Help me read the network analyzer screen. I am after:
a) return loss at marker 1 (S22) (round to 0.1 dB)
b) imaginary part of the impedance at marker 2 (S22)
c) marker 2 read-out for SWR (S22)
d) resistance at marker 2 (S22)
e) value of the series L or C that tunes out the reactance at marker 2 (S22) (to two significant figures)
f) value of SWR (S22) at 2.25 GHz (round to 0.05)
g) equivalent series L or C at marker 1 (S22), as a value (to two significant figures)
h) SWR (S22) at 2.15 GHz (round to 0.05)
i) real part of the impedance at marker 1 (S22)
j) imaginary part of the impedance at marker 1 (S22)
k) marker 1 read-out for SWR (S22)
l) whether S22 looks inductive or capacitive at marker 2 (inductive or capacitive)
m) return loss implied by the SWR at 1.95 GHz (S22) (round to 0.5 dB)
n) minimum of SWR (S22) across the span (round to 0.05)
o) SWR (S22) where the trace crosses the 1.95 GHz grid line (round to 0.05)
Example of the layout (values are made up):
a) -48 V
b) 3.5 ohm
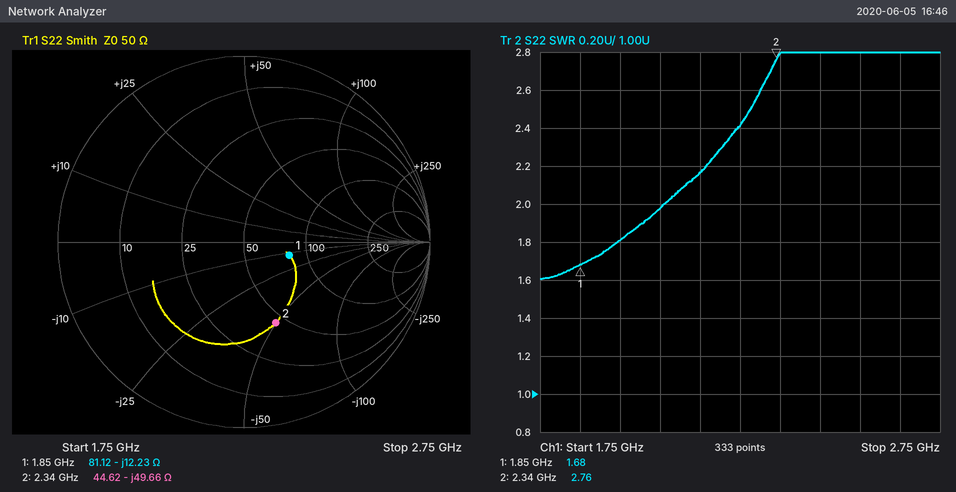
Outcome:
a) 11.9 dB
b) -49.66 Ω
c) 2.76
d) 44.62 Ω
e) 3.4 nH
f) 2.40
g) 7.0 pF
h) 2.15
i) 81.12 Ω
j) -12.23 Ω
k) 1.68
l) capacitive
m) 11.0 dB
n) 1.60
o) 1.80
